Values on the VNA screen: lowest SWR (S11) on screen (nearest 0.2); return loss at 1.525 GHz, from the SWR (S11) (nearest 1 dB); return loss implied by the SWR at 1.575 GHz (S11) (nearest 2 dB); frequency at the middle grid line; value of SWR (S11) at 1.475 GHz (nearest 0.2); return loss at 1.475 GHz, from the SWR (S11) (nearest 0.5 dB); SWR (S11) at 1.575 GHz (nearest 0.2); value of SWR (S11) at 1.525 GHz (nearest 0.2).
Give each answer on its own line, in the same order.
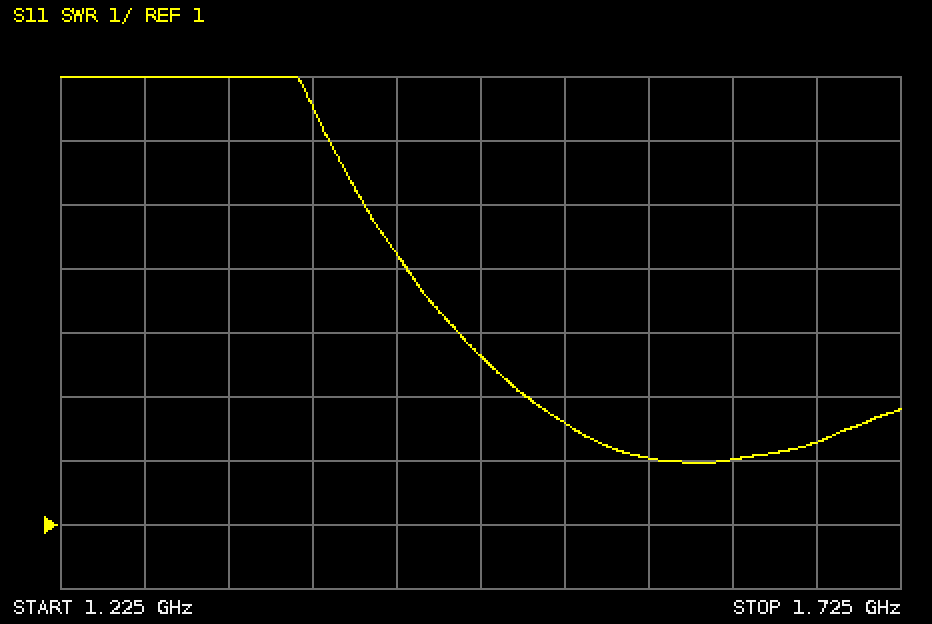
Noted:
2.0
7 dB
10 dB
1.475 GHz
3.6
5.0 dB
2.0
2.6
